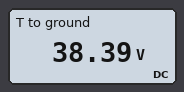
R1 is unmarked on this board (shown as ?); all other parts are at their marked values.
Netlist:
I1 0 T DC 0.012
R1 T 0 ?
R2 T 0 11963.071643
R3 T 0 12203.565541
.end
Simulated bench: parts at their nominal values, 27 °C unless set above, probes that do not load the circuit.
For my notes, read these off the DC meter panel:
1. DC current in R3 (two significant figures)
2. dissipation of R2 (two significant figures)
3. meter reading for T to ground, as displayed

3.1 mA
120 mW
38.39 V
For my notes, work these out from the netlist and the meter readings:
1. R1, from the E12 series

6.8 kΩ
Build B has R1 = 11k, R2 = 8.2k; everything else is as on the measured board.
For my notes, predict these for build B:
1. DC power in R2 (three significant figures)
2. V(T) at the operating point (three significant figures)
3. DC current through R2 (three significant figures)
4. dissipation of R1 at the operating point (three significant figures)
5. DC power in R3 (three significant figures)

202 mW
40.7 V
4.96 mA
151 mW
136 mW
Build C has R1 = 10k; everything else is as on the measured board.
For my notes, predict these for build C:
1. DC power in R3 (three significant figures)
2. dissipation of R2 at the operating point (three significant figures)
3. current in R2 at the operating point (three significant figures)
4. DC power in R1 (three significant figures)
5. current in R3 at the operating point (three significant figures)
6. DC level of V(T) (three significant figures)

167 mW
171 mW
3.78 mA
204 mW
3.70 mA
45.2 V
